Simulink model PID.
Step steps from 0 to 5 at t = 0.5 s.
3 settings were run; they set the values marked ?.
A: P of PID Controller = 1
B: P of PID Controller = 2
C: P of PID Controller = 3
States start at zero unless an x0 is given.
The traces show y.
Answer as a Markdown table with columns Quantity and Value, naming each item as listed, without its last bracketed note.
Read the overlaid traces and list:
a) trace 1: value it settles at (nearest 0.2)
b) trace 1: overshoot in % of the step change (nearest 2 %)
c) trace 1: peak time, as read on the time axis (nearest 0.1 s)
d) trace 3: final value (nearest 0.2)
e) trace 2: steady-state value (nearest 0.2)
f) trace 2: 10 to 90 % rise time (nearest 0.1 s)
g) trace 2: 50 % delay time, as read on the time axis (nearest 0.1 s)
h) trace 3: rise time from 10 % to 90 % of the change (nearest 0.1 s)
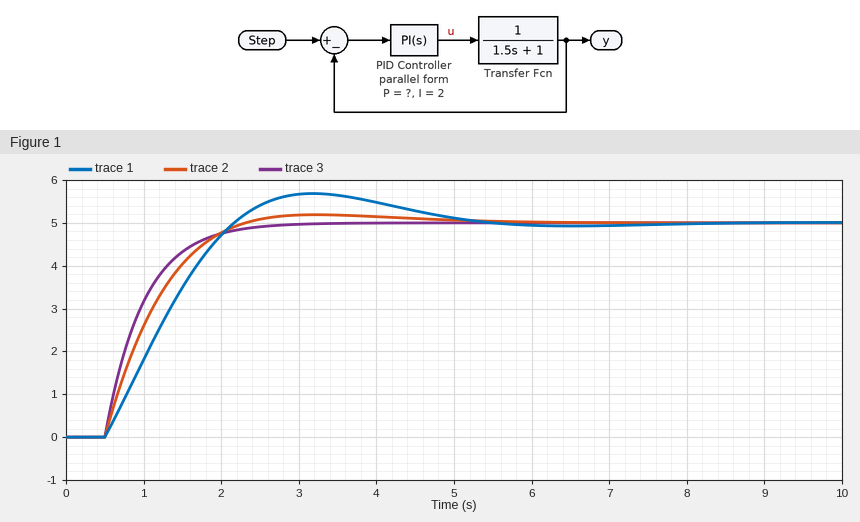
| Quantity | Value |
|---|---|
| trace 1: value it settles at | 5.0 |
| trace 1: overshoot in % of the step change | 14 % |
| trace 1: peak time, as read on the time axis | 3.2 s |
| trace 3: final value | 5.0 |
| trace 2: steady-state value | 5.0 |
| trace 2: 10 to 90 % rise time | 1.2 s |
| trace 2: 50 % delay time, as read on the time axis | 1.0 s |
| trace 3: rise time from 10 % to 90 % of the change | 1.1 s |
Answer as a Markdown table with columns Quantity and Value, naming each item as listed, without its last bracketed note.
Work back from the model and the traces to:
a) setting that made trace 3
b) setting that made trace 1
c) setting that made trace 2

| Quantity | Value |
|---|---|
| setting that made trace 3 | C |
| setting that made trace 1 | A |
| setting that made trace 2 | B |
